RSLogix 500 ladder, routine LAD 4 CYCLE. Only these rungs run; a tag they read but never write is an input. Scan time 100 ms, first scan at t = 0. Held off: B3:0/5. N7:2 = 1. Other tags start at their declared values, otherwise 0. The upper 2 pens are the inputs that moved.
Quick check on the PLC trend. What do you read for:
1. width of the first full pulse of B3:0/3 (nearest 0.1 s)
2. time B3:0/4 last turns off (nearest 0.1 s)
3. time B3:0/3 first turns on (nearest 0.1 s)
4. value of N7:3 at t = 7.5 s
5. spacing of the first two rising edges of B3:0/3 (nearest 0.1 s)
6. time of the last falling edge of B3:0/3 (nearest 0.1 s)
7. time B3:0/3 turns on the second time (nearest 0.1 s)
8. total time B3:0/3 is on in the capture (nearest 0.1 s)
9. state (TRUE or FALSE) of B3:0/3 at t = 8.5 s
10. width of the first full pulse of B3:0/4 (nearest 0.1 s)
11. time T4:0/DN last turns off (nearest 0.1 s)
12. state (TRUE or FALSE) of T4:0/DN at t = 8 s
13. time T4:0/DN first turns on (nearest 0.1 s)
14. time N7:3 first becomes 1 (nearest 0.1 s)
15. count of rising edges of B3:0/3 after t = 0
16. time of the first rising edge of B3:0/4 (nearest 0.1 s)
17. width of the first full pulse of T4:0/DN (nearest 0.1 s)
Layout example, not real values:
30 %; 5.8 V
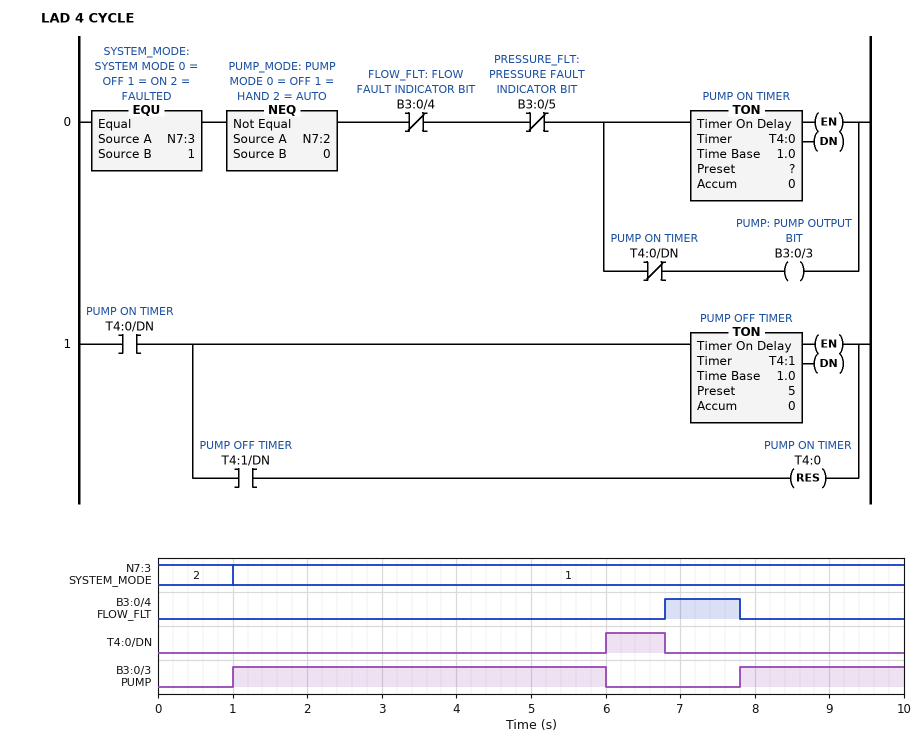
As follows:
5.0 s; 7.8 s; 1.0 s; 1; 6.8 s; 6.0 s; 7.8 s; 7.2 s; TRUE; 1.0 s; 6.8 s; FALSE; 6.0 s; 1.0 s; 2; 6.8 s; 0.8 s
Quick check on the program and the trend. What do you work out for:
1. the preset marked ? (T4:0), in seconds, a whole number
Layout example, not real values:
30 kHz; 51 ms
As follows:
5 s
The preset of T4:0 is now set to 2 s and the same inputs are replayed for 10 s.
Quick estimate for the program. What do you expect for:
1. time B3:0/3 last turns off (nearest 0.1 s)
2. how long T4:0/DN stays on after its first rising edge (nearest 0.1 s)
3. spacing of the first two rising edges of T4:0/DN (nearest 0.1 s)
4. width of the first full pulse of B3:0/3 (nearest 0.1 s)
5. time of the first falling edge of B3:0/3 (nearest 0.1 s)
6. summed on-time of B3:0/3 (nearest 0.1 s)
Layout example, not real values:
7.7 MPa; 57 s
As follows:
9.8 s; 3.8 s; 6.8 s; 2.0 s; 3.0 s; 4.0 s
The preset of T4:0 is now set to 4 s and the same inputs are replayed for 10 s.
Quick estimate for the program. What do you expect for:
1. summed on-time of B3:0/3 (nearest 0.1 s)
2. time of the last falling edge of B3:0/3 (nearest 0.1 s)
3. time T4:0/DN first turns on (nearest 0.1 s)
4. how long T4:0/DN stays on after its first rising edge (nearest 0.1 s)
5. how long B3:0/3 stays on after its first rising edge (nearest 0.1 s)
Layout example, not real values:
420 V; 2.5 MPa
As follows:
6.2 s; 5.0 s; 5.0 s; 1.8 s; 4.0 s
